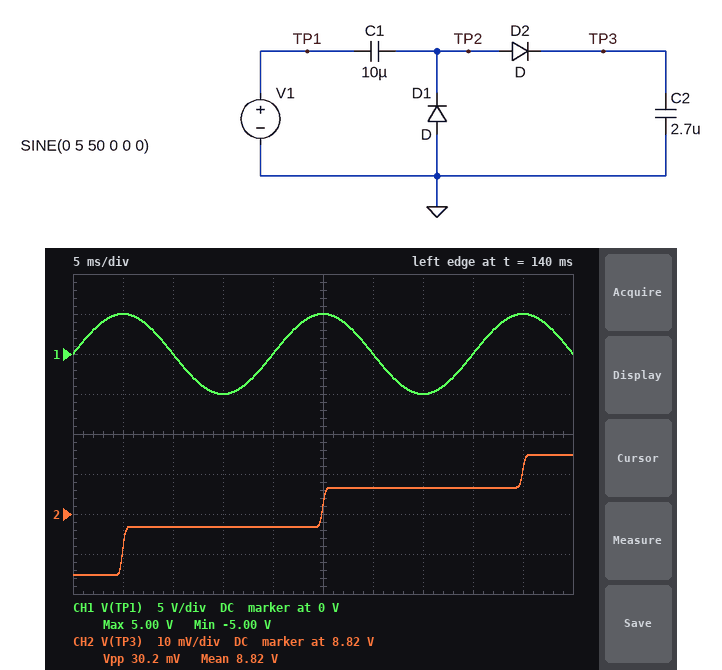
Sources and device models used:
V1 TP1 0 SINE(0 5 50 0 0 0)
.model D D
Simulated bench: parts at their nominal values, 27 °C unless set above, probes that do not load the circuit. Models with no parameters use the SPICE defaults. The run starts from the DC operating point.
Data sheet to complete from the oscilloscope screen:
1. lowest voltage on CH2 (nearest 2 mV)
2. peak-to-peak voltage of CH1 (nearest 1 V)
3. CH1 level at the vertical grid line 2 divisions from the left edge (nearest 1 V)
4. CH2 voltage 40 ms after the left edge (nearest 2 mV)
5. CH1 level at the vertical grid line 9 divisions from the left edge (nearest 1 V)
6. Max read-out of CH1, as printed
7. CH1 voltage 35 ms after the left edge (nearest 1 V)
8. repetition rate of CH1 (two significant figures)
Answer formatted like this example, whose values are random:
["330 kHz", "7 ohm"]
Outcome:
["8.804 V", "10 V", "0 V", "8.826 V", "5 V", "5.00 V", "-5 V", "50 Hz"]
